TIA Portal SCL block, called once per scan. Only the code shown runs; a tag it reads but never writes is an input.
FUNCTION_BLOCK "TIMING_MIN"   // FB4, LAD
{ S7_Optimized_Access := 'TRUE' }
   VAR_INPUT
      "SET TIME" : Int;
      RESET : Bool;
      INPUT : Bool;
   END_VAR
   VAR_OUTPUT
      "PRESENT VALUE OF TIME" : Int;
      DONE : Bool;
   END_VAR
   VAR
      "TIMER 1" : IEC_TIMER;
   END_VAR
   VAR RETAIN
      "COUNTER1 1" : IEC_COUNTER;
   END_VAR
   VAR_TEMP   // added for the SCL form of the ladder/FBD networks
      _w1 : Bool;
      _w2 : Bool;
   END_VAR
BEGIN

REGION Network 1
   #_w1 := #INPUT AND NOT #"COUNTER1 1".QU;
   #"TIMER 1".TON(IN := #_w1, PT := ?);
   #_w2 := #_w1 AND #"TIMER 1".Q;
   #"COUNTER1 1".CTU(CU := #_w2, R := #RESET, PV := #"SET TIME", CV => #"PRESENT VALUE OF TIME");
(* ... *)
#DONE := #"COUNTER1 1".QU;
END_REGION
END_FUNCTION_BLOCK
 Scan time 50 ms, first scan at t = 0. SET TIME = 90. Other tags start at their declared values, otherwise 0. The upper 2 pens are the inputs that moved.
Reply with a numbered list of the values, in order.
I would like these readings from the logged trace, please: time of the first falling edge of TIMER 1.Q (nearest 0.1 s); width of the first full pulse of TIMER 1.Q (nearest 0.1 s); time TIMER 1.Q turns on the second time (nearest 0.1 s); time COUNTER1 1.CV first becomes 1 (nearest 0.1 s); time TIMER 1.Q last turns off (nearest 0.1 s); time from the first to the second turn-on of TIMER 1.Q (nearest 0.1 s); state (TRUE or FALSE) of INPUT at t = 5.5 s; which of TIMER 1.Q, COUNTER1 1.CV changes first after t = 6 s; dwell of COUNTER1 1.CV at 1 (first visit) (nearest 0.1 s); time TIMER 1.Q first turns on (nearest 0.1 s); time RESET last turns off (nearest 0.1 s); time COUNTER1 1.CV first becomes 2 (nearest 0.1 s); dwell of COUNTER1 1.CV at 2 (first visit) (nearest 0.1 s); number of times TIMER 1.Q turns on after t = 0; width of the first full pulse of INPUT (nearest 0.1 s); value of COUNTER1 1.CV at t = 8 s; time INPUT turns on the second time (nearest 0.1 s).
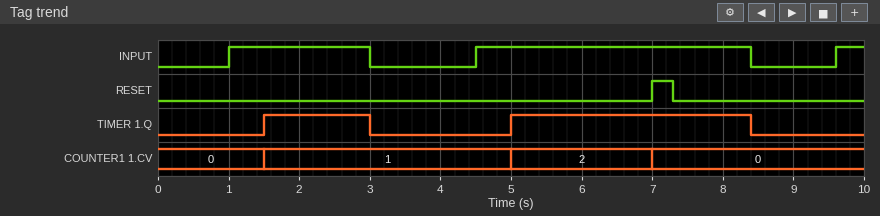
1. 3.0 s
2. 1.5 s
3. 5.0 s
4. 1.5 s
5. 8.4 s
6. 3.5 s
7. TRUE
8. COUNTER1 1.CV
9. 3.5 s
10. 1.5 s
11. 7.3 s
12. 5.0 s
13. 2.0 s
14. 2
15. 2.0 s
16. 0
17. 4.5 s
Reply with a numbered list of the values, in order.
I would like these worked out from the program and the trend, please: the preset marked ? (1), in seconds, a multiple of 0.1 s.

1. 0.5 s
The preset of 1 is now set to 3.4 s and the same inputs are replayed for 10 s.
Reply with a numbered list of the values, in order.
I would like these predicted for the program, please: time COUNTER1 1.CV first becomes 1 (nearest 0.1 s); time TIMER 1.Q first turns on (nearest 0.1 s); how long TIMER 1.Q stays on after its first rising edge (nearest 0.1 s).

1. 7.9 s
2. 7.9 s
3. 0.5 s
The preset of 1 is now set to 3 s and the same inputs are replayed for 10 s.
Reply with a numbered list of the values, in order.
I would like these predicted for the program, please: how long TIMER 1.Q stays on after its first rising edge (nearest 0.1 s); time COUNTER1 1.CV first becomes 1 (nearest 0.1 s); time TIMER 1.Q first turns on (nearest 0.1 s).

1. 0.9 s
2. 7.5 s
3. 7.5 s
